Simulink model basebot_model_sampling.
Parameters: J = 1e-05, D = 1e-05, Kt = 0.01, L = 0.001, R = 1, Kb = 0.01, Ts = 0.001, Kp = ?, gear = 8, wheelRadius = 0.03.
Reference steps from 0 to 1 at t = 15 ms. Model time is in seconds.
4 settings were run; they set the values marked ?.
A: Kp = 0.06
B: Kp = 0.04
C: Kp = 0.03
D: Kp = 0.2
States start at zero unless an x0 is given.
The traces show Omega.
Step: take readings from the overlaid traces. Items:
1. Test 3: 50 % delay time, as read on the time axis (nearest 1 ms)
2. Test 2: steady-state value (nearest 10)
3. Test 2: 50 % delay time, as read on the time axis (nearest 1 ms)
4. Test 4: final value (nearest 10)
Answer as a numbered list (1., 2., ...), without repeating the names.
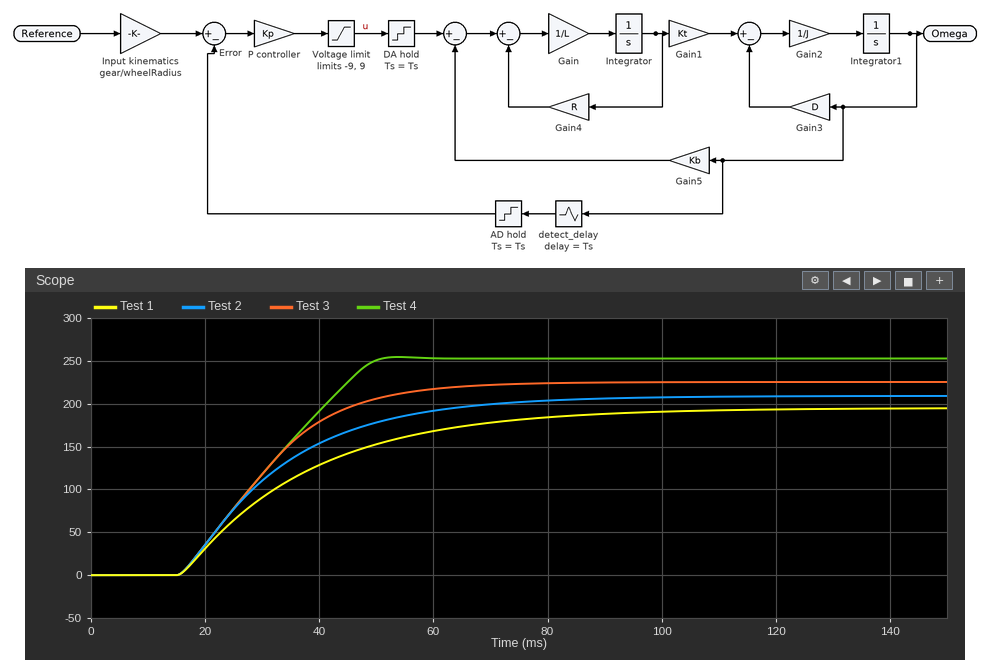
1. 29 ms
2. 210
3. 29 ms
4. 250
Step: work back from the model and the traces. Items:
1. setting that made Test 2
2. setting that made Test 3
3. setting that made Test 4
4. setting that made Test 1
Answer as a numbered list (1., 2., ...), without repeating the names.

1. B
2. A
3. D
4. C
